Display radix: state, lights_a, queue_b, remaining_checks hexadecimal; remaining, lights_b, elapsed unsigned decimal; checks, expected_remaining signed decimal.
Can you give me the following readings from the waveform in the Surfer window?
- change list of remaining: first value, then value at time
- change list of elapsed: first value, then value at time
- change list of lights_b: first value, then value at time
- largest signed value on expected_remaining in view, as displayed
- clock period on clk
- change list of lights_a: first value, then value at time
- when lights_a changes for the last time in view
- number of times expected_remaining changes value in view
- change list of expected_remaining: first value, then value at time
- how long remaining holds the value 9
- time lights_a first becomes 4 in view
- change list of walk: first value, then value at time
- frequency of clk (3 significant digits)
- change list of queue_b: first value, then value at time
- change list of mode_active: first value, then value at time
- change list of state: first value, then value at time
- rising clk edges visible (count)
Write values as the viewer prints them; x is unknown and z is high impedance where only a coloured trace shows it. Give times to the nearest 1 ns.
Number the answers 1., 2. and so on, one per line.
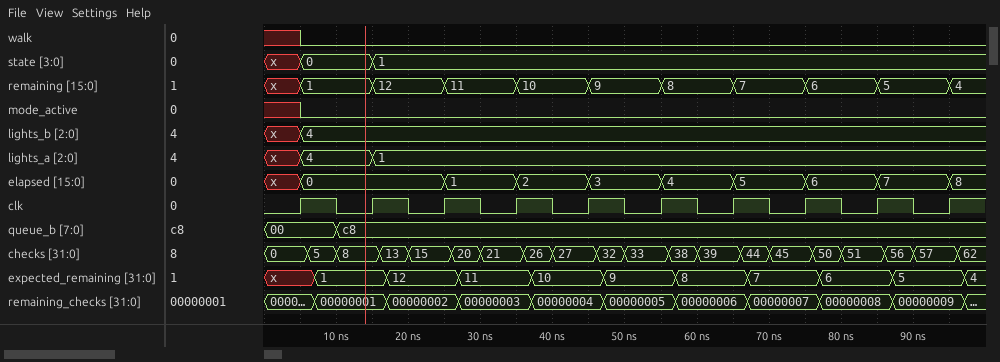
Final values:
1. x, 1 at 5 ns, 12 at 15 ns, 11 at 25 ns, 10 at 35 ns, 9 at 45 ns, 8 at 55 ns, 7 at 65 ns, 6 at 75 ns, 5 at 85 ns, 4 at 95 ns
2. x, 0 at 5 ns, 1 at 25 ns, 2 at 35 ns, 3 at 45 ns, 4 at 55 ns, 5 at 65 ns, 6 at 75 ns, 7 at 85 ns, 8 at 95 ns
3. x, 4 at 5 ns
4. 12
5. 10 ns
6. x, 4 at 5 ns, 1 at 15 ns
7. 15 ns
8. 10
9. x, 1 at 7 ns, 12 at 17 ns, 11 at 27 ns, 10 at 37 ns, 9 at 47 ns, 8 at 57 ns, 7 at 67 ns, 6 at 77 ns, 5 at 87 ns, 4 at 97 ns
10. 10 ns
11. 5 ns
12. x, 0 at 5 ns
13. 100 MHz
14. 00, c8 at 10 ns
15. x, 0 at 5 ns
16. x, 0 at 5 ns, 1 at 15 ns
17. 10
